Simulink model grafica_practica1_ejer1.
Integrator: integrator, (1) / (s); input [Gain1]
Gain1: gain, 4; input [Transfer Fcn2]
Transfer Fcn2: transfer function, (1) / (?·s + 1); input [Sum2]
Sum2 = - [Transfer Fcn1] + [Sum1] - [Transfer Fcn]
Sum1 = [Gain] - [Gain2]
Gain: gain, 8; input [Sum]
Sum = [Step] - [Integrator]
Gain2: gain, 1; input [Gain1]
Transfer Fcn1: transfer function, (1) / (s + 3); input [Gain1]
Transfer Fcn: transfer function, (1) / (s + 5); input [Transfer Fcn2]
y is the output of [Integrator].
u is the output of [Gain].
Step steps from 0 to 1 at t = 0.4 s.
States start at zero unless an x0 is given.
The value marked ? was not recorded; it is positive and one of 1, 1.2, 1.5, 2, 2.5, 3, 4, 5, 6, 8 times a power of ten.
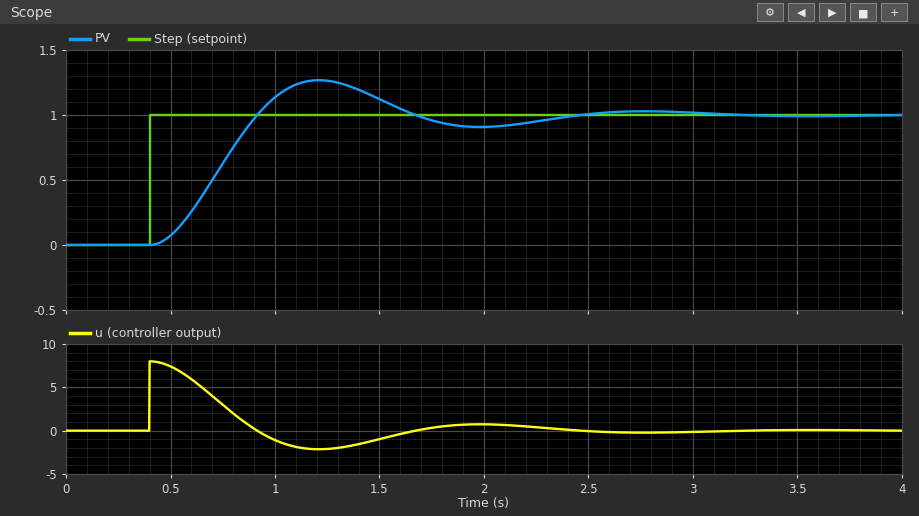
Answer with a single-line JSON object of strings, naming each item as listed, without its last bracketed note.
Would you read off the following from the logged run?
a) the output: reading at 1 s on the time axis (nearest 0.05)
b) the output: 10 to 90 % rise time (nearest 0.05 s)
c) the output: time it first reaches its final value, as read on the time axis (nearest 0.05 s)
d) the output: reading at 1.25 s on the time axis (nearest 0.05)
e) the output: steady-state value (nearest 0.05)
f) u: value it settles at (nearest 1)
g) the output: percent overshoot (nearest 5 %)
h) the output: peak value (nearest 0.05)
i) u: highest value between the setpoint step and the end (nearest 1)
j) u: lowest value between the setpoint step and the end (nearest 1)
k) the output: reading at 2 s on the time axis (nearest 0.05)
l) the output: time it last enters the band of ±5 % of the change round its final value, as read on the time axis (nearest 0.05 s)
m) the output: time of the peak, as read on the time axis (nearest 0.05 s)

{"the output: reading at 1 s on the time axis": "1.15", "the output: 10 to 90 % rise time": "0.35 s", "the output: time it first reaches its final value, as read on the time axis": "0.90 s", "the output: reading at 1.25 s on the time axis": "1.25", "the output: steady-state value": "1.00", "u: value it settles at": "0", "the output: percent overshoot": "25 %", "the output: peak value": "1.25", "u: highest value between the setpoint step and the end": "8", "u: lowest value between the setpoint step and the end": "-2", "the output: reading at 2 s on the time axis": "0.90", "the output: time it last enters the band of ±5 % of the change round its final value, as read on the time axis": "2.25 s", "the output: time of the peak, as read on the time axis": "1.20 s"}
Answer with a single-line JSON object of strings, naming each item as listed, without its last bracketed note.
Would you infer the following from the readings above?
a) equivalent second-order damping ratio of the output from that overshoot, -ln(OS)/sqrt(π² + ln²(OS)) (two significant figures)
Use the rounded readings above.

{"equivalent second-order damping ratio of the output from that overshoot, -ln(OS)/sqrt(π² + ln²(OS))": "0.40"}
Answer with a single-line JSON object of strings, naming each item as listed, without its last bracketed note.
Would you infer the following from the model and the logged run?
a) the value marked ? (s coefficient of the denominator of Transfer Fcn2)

{"the value marked ?": "2"}
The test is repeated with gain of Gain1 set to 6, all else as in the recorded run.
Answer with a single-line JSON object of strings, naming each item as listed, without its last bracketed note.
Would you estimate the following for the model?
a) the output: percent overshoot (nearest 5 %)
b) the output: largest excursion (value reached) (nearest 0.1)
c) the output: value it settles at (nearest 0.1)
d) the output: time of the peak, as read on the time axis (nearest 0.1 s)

{"the output: percent overshoot": "20 %", "the output: largest excursion (value reached)": "1.2", "the output: value it settles at": "1.0", "the output: time of the peak, as read on the time axis": "1.1 s"}
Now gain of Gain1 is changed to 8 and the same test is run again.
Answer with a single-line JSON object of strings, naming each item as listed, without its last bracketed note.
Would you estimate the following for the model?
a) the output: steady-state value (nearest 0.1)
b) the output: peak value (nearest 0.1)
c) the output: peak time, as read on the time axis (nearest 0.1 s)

{"the output: steady-state value": "1.0", "the output: peak value": "1.2", "the output: peak time, as read on the time axis": "1.0 s"}
